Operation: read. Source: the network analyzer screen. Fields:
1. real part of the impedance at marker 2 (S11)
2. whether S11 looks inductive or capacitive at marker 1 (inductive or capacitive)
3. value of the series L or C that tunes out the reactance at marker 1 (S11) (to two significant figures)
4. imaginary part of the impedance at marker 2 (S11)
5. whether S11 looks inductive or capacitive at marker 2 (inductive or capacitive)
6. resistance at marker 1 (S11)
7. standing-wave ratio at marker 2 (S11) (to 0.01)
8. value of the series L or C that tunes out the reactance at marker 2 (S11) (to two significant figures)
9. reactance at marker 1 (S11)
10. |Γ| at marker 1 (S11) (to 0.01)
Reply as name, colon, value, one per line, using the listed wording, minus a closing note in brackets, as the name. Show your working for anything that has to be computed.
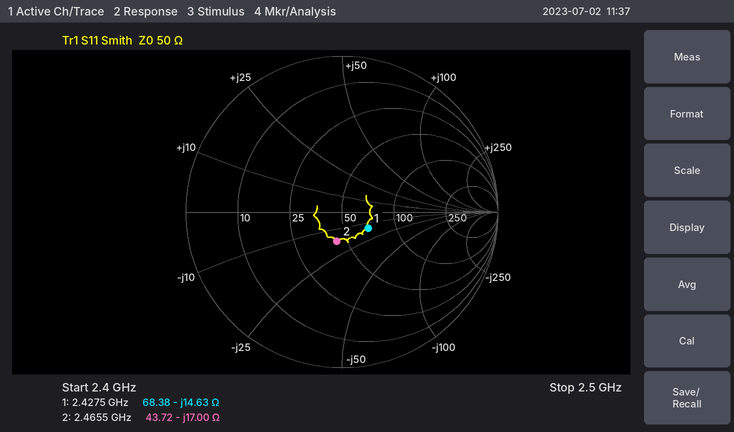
real part of the impedance at marker 2: 43.72 Ω
whether S11 looks inductive or capacitive at marker 1: capacitive
value of the series L or C that tunes out the reactance at marker 1 (S11): L = 14.63 Ω/(2π × 2.4275 GHz) ≈ 959 pH, so 960 pH to two significant figures
imaginary part of the impedance at marker 2: -17.00 Ω
whether S11 looks inductive or capacitive at marker 2: capacitive
resistance at marker 1: 68.38 Ω
standing-wave ratio at marker 2 (S11): 1.47
value of the series L or C that tunes out the reactance at marker 2 (S11): L = 17 Ω/(2π × 2.4655 GHz) ≈ 1.1 nH
reactance at marker 1: -14.63 Ω
|Γ| at marker 1 (S11): 0.20
